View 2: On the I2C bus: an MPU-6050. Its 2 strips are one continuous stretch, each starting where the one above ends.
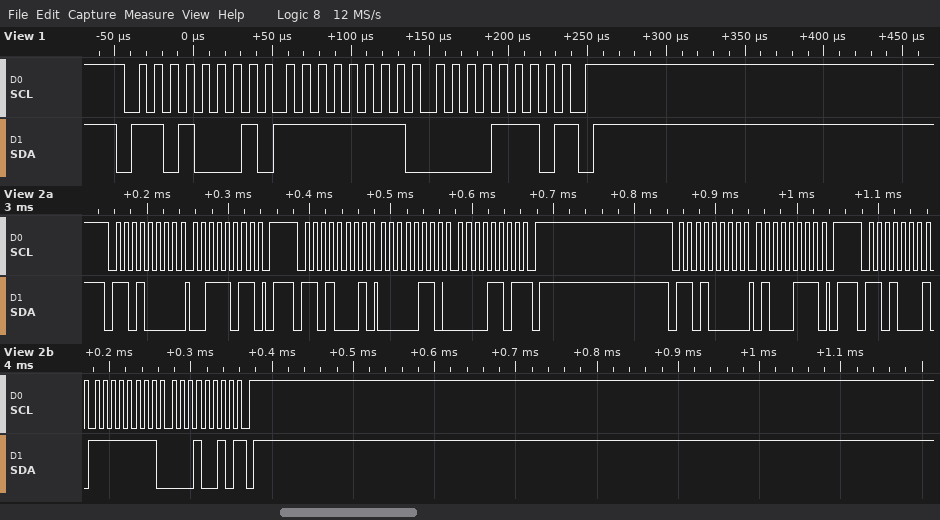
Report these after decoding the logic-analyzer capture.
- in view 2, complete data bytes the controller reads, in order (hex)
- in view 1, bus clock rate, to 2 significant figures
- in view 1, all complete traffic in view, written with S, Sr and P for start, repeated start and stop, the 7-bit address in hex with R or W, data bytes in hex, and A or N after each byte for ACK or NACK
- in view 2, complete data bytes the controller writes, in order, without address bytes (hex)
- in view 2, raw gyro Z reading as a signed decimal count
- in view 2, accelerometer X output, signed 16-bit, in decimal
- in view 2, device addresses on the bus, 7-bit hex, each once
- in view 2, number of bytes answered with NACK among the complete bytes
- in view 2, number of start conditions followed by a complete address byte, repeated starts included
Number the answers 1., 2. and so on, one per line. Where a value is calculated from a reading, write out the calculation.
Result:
1. 06 0D FF 12
2. 100 kHz
3. S 68R A FF A 0E N P
4. 3B 47
5. 0xFF12 = -238
6. 0x060D = 1549
7. 0x68
8. 2
9. 4
